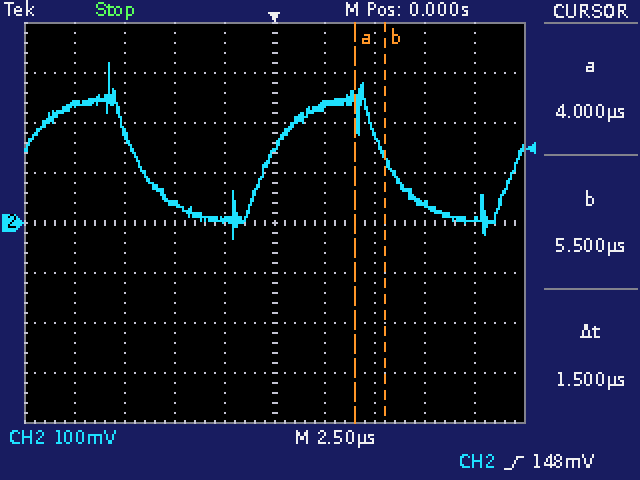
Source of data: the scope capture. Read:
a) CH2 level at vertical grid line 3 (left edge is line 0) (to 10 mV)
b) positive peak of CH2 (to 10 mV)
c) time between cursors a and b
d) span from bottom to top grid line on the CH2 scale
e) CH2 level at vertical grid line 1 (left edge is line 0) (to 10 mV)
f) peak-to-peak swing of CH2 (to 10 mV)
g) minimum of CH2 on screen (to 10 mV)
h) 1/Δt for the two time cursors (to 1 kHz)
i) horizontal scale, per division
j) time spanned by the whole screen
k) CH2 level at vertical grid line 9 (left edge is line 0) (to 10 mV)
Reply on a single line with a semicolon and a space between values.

40 mV; 320 mV; 1.5 µs; 800 mV; 240 mV; 350 mV; -30 mV; 667 kHz; 2.5 µs; 25 µs; 10 mV
